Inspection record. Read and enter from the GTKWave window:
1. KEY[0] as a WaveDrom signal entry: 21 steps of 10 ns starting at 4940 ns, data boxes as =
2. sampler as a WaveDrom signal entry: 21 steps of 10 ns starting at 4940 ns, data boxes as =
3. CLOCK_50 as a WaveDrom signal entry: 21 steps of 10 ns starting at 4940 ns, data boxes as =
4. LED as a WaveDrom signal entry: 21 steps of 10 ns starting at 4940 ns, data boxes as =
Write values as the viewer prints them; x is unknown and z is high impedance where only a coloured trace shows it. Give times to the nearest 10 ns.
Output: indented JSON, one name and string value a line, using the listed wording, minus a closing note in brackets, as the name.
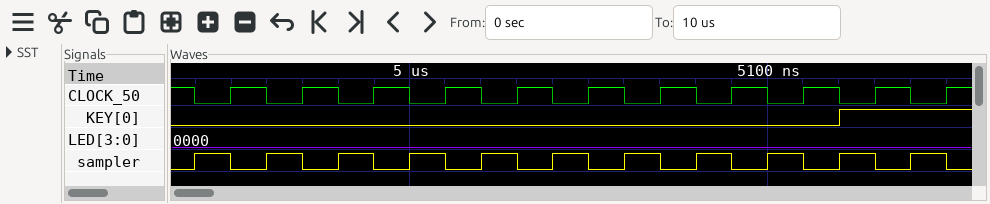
{
  "KEY[0] as a WaveDrom signal entry: 21 steps of 10 ns starting at 4940 ns, data boxes as =": "{name: 'KEY[0]', wave: '0.................1..'}",
  "sampler as a WaveDrom signal entry: 21 steps of 10 ns starting at 4940 ns, data boxes as =": "{name: 'sampler', wave: '101010101010101010101'}",
  "CLOCK_50 as a WaveDrom signal entry: 21 steps of 10 ns starting at 4940 ns, data boxes as =": "{name: 'CLOCK_50', wave: '010101010101010101010'}",
  "LED as a WaveDrom signal entry: 21 steps of 10 ns starting at 4940 ns, data boxes as =": "{name: 'LED', wave: '=....................', data: '0000'}"
}
